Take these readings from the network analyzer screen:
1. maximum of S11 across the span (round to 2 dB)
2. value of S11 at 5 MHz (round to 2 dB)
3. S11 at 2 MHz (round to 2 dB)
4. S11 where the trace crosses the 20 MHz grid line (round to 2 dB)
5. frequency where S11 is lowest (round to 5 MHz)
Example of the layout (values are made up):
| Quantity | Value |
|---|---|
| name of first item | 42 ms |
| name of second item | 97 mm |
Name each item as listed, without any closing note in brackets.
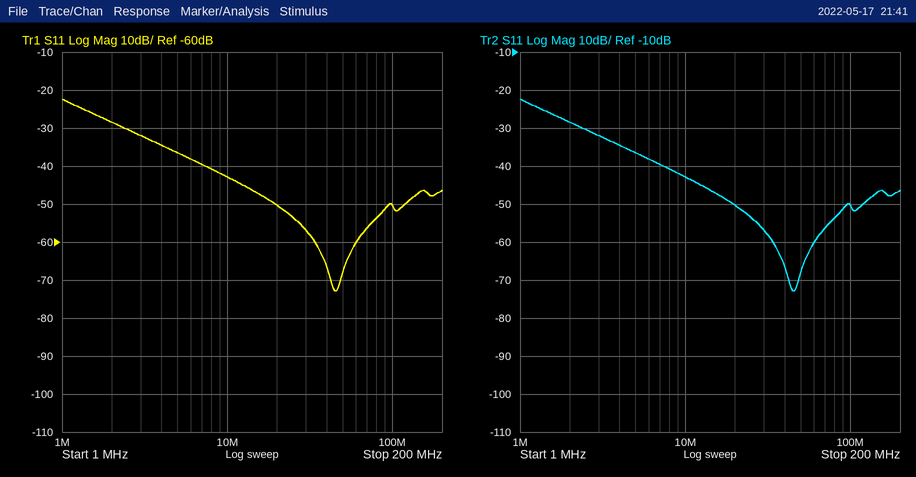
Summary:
| Quantity | Value |
|---|---|
| maximum of S11 across the span | -22 dB |
| value of S11 at 5 MHz | -36 dB |
| S11 at 2 MHz | -28 dB |
| S11 where the trace crosses the 20 MHz grid line | -50 dB |
| frequency where S11 is lowest | 45 MHz |
